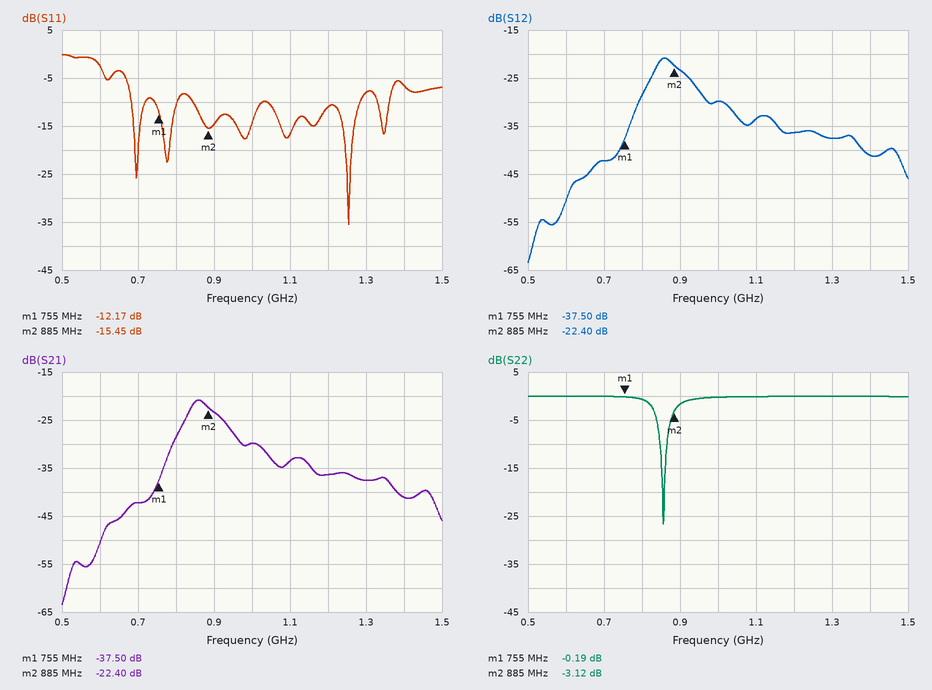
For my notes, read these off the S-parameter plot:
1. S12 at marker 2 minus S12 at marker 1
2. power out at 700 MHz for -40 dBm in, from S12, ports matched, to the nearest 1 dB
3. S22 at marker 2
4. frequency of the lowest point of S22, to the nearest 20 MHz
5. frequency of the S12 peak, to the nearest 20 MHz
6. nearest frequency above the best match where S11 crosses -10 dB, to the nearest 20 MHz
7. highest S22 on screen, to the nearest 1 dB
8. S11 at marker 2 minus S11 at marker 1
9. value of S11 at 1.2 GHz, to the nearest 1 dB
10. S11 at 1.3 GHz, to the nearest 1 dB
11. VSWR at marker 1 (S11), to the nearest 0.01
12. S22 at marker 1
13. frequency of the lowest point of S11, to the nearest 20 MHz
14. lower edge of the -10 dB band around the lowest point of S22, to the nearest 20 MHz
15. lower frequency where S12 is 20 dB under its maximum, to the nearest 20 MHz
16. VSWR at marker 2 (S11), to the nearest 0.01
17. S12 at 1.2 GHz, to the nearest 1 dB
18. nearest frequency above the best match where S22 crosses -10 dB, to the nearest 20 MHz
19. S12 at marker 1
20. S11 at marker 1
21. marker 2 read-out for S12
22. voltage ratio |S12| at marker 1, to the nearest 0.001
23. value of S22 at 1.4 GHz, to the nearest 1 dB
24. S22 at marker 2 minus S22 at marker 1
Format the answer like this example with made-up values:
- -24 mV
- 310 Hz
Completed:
- 15.10 dB
- -82 dBm
- -3.12 dB
- 860 MHz
- 860 MHz
- 1.28 GHz
- 0 dB
- -3.28 dB
- -11 dB
- -8 dB
- 1.65
- -0.19 dB
- 1.26 GHz
- 840 MHz
- 740 MHz
- 1.41
- -36 dB
- 860 MHz
- -37.50 dB
- -12.17 dB
- -22.40 dB
- 0.013
- 0 dB
- -2.93 dB
